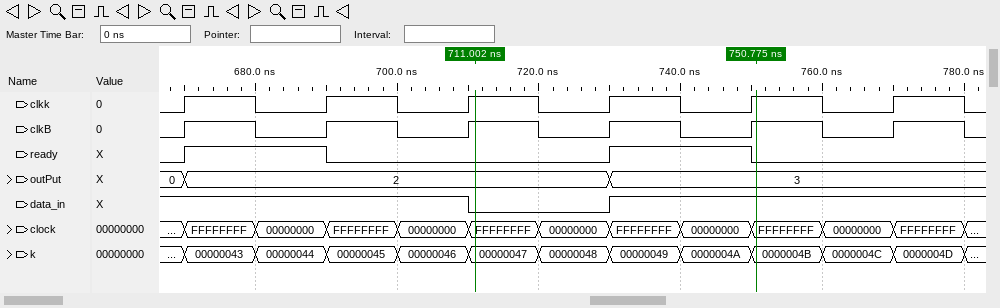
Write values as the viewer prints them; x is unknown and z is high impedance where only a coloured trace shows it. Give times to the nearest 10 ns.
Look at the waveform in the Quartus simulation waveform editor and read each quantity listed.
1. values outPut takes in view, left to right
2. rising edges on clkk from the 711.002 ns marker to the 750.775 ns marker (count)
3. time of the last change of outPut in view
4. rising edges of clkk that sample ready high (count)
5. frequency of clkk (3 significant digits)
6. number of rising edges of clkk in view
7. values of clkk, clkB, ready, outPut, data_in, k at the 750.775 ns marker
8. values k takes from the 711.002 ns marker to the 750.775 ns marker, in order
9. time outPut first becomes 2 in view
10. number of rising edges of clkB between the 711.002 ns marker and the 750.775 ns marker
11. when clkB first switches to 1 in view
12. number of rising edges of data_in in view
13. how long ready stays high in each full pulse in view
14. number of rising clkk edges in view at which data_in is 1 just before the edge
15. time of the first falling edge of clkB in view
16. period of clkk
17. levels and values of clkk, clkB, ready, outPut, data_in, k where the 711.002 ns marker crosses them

0, 2, 3
2
730 ns
2
50.0 MHz
6
clkk=1, clkB=1, ready=0, outPut=3, data_in=1, k=0000004B
00000047, 00000048, 00000049, 0000004A, 0000004B
670 ns
2
670 ns
1
20 ns, 20 ns
5
680 ns
20 ns
clkk=1, clkB=1, ready=0, outPut=2, data_in=0, k=00000047
